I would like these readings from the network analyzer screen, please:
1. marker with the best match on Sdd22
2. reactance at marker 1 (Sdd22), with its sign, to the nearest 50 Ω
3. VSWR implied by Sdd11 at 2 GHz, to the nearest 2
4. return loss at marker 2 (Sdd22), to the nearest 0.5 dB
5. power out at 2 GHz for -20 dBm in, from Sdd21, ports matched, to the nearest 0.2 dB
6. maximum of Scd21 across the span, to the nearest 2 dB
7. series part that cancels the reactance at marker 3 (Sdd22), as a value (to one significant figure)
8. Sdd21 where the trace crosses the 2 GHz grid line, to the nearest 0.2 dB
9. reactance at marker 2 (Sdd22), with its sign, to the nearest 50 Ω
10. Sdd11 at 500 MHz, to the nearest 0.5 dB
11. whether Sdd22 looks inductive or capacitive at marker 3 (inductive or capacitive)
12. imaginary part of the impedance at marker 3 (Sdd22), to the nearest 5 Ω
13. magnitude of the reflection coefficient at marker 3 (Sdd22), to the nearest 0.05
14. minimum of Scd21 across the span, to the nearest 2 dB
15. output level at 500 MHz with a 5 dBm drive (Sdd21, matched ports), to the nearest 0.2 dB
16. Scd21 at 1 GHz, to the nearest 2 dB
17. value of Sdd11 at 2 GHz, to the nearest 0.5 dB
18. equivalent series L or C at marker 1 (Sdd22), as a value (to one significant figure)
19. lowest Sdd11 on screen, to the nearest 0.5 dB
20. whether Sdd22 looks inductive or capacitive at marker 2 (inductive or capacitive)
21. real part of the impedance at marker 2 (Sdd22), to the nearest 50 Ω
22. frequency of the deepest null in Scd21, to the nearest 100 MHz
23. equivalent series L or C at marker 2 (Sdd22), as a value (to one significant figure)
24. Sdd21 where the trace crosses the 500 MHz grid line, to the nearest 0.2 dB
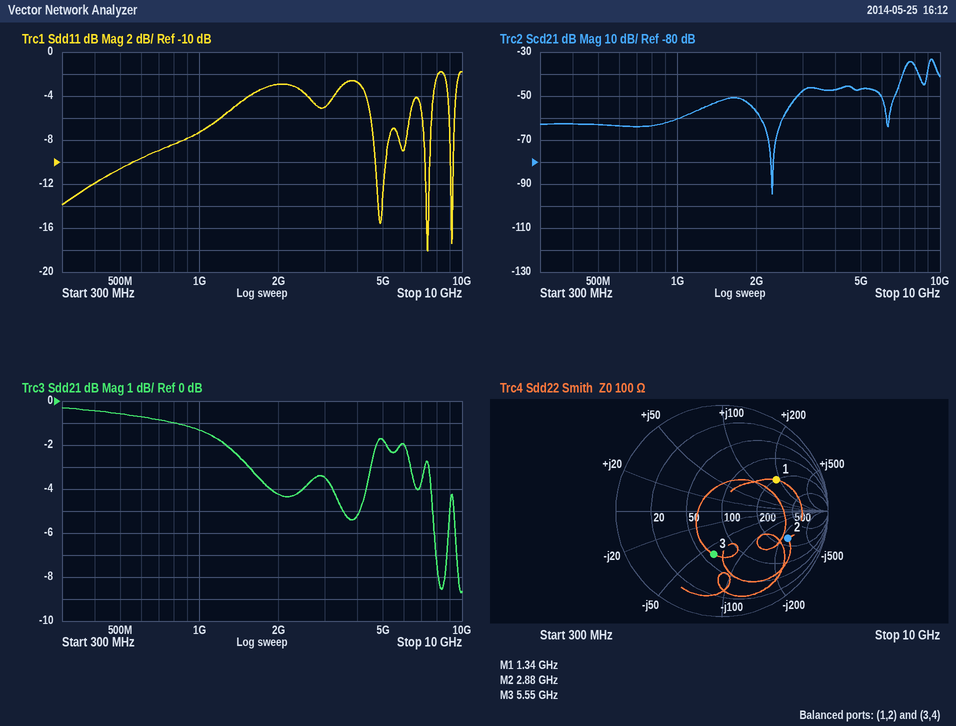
marker 3
+200 Ω
6
3.5 dB
-24.2 dBm
-34 dB
2 nH
-4.2 dB
-250 Ω
-10.5 dB
capacitive
-60 Ω
0.40
-94 dB
4.4 dBm
-60 dB
-3.0 dB
20 nH
-18.0 dB
capacitive
250 Ω
2.3 GHz
200 fF
-0.6 dB
